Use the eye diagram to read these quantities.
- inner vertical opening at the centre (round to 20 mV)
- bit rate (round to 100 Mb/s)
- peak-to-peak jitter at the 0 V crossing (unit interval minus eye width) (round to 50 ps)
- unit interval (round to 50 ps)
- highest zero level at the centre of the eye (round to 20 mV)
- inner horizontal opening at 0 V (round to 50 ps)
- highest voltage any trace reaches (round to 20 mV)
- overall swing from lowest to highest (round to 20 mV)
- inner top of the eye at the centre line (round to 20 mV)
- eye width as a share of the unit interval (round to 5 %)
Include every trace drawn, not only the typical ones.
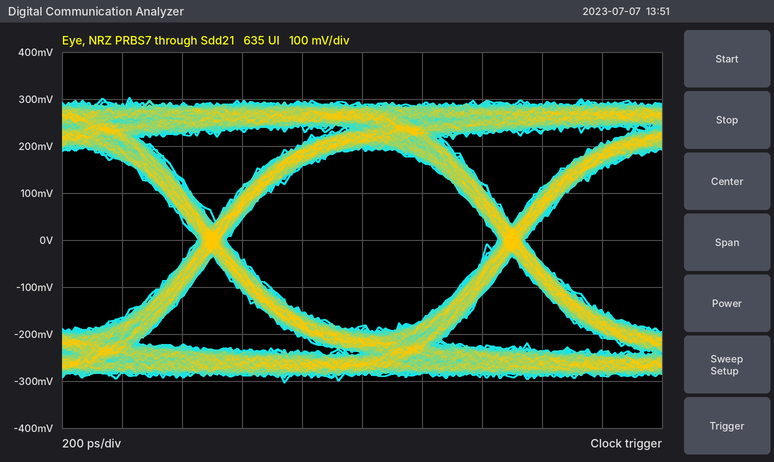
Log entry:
380 mV
1.0 Gb/s
100 ps
1.00 ns
-180 mV
900 ps
300 mV
600 mV
200 mV
90 %
